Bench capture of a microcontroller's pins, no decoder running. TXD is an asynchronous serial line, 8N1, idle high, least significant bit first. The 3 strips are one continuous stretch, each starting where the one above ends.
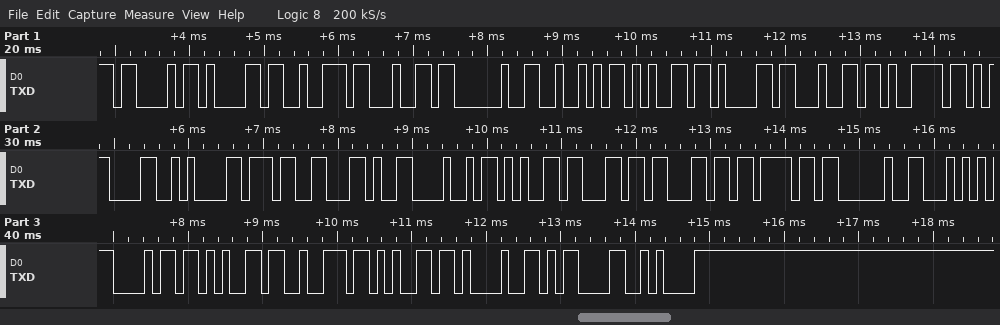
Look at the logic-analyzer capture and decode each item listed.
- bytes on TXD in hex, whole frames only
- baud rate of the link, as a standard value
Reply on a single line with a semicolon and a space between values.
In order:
43 61 72 64 20 52 65 61 64 79 0D 0A 37 2C 48 65 6C 6C 6F 20 54 68 65 72 65 21 0D 0A; 9600 baud
